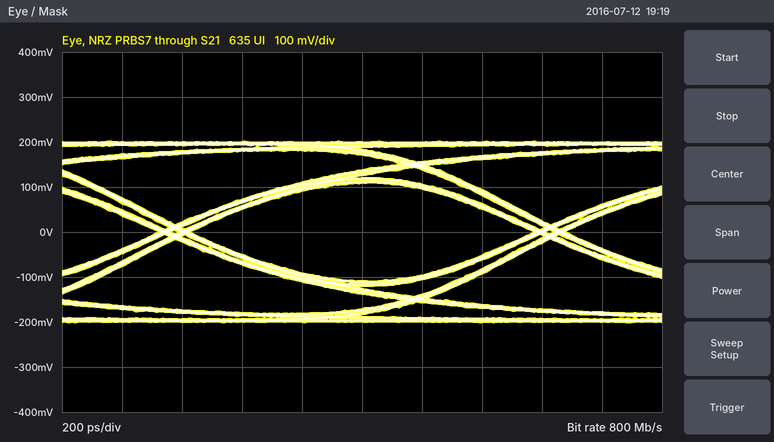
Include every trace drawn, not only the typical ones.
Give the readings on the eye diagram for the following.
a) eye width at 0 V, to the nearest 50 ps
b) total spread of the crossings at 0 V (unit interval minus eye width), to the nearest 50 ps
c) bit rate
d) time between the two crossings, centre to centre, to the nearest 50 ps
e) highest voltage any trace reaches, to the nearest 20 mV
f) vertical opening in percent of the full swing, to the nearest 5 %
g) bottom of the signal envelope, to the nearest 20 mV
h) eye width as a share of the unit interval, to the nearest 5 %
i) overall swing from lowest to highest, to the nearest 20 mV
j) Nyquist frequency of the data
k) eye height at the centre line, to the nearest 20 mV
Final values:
1.15 ns
100 ps
800 Mb/s
1.25 ns
200 mV
55 %
-200 mV
90 %
400 mV
400 MHz
220 mV
